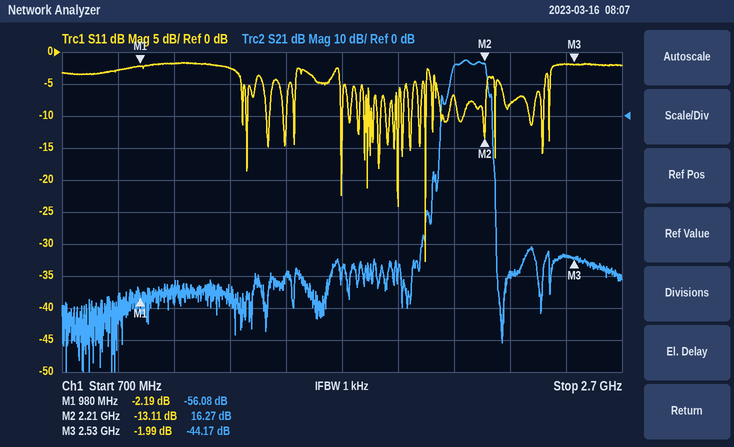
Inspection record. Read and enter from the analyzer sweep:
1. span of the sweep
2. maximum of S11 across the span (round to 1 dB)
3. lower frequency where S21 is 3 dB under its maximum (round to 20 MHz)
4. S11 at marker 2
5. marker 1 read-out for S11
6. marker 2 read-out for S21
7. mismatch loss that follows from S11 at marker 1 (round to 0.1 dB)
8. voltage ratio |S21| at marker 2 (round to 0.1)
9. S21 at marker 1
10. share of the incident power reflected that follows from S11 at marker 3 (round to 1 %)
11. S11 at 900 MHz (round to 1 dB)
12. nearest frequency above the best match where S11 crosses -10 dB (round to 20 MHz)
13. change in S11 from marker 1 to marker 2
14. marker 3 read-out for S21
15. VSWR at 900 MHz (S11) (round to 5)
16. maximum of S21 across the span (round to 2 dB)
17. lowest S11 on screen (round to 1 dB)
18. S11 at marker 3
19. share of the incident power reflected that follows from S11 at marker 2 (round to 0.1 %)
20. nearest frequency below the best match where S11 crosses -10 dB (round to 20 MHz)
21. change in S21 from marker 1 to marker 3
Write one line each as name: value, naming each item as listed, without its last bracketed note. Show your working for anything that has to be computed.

span of the sweep: 2 GHz
maximum of S11 across the span: -2 dB
lower frequency where S21 is 3 dB under its maximum: 2.10 GHz
S11 at marker 2: -13.11 dB
marker 1 read-out for S11: -2.19 dB
marker 2 read-out for S21: 16.27 dB
mismatch loss that follows from S11 at marker 1: −10 log10(1 − 10^(-2.19/10)) ≈ 4.0 dB
voltage ratio |S21| at marker 2: 10^(16.27/20) ≈ 6.5
S21 at marker 1: -56.08 dB
share of the incident power reflected that follows from S11 at marker 3: 10^(-1.99/10) ≈ 63 %
S11 at 900 MHz: -3 dB
nearest frequency above the best match where S11 crosses -10 dB: 2.00 GHz
change in S11 from marker 1 to marker 2: -13.11 − (-2.19) = -10.92 dB
marker 3 read-out for S21: -44.17 dB
VSWR at 900 MHz (S11): |Γ| = 10^(-3/20) = 0.7079; VSWR = (1 + 0.7079)/(1 − 0.7079) ≈ 5.85, so 5 to the nearest 5
maximum of S21 across the span: 18 dB
lowest S11 on screen: -33 dB
S11 at marker 3: -1.99 dB
share of the incident power reflected that follows from S11 at marker 2: 10^(-13.11/10) ≈ 4.9 %
nearest frequency below the best match where S11 crosses -10 dB: 2.00 GHz
change in S21 from marker 1 to marker 3: -44.17 − (-56.08) = 11.91 dB
